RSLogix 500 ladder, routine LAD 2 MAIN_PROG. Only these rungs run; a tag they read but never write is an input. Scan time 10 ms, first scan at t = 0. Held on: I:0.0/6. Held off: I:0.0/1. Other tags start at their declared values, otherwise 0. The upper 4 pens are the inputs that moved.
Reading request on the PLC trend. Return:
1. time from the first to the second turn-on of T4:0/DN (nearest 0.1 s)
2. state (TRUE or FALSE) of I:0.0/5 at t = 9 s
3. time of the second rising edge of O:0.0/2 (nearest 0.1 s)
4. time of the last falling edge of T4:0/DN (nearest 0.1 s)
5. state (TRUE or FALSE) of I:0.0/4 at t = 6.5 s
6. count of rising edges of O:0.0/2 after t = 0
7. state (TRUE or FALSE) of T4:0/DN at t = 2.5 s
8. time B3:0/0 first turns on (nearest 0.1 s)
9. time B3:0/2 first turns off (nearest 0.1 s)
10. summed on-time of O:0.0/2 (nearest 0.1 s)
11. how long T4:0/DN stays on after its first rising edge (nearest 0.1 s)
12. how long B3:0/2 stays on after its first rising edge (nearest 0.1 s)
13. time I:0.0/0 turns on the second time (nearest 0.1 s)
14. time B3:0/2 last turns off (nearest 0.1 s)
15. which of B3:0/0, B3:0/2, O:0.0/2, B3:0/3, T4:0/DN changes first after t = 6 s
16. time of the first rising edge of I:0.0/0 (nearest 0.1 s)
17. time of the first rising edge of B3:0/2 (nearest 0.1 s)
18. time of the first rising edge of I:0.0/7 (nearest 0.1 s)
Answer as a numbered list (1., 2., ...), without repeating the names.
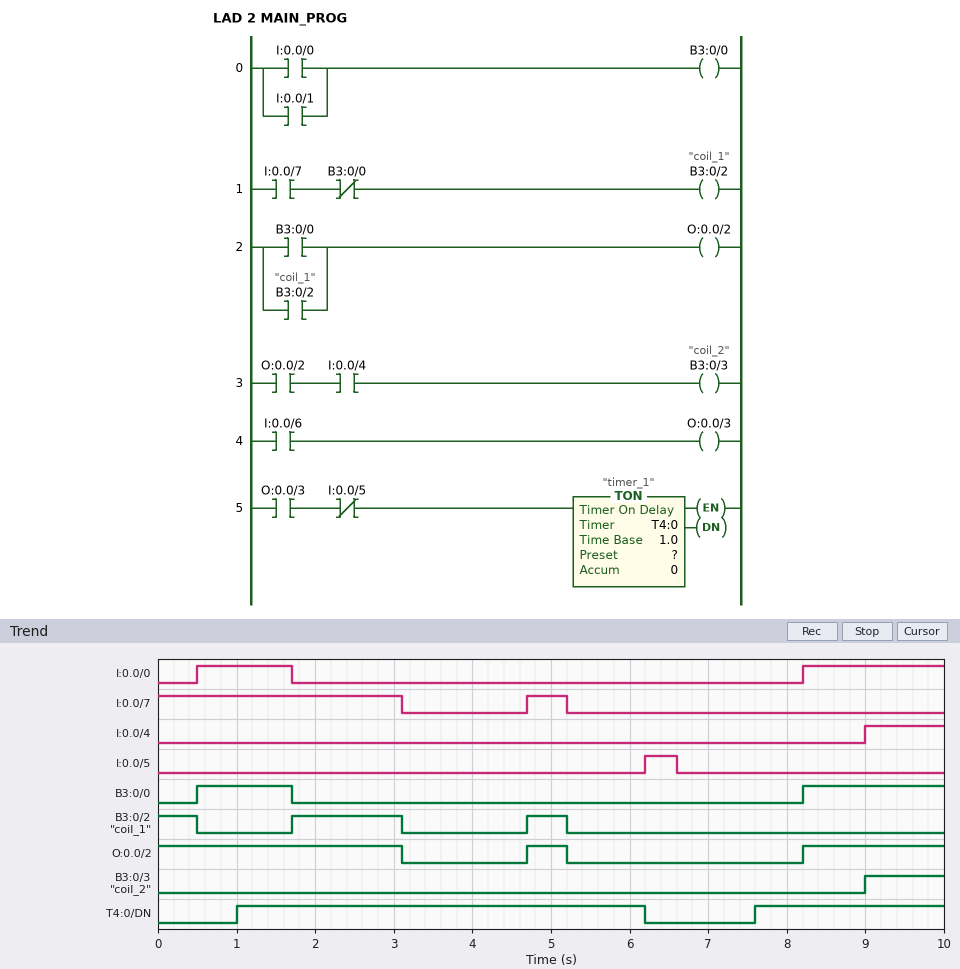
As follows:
1. 6.6 s
2. FALSE
3. 8.2 s
4. 6.2 s
5. FALSE
6. 2
7. TRUE
8. 0.5 s
9. 0.5 s
10. 5.4 s
11. 5.2 s
12. 1.4 s
13. 8.2 s
14. 5.2 s
15. T4:0/DN
16. 0.5 s
17. 1.7 s
18. 4.7 s
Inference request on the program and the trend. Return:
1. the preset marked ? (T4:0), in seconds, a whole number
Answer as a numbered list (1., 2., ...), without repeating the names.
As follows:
1. 1 s
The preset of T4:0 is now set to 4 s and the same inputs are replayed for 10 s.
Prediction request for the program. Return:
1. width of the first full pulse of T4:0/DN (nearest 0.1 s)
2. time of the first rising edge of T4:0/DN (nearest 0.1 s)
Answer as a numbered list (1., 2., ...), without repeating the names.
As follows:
1. 2.2 s
2. 4.0 s
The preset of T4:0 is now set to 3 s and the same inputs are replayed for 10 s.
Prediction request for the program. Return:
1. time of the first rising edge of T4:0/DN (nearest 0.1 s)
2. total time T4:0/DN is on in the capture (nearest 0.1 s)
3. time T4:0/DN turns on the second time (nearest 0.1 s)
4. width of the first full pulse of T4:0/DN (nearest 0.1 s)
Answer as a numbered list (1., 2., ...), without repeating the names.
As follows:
1. 3.0 s
2. 3.6 s
3. 9.6 s
4. 3.2 s
